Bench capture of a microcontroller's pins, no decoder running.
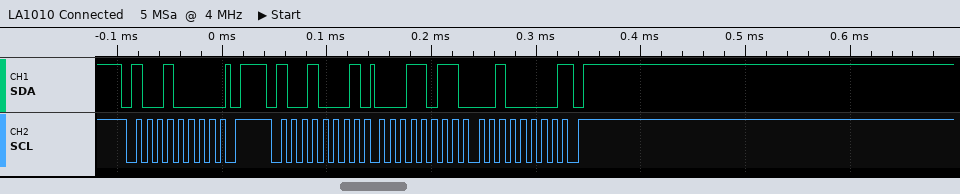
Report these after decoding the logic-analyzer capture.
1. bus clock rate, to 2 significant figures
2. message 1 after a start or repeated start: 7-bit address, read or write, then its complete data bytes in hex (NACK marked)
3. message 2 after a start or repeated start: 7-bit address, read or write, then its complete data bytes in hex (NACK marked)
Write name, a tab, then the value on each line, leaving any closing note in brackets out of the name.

bus clock rate, to 2 significant figures	100 kHz
message 1 after a start or repeated start: 7-bit address, read or write, then its complete data bytes in hex	0x48 write
message 2 after a start or repeated start: 7-bit address, read or write, then its complete data bytes in hex	0x48 read: 1B 20 NACK
